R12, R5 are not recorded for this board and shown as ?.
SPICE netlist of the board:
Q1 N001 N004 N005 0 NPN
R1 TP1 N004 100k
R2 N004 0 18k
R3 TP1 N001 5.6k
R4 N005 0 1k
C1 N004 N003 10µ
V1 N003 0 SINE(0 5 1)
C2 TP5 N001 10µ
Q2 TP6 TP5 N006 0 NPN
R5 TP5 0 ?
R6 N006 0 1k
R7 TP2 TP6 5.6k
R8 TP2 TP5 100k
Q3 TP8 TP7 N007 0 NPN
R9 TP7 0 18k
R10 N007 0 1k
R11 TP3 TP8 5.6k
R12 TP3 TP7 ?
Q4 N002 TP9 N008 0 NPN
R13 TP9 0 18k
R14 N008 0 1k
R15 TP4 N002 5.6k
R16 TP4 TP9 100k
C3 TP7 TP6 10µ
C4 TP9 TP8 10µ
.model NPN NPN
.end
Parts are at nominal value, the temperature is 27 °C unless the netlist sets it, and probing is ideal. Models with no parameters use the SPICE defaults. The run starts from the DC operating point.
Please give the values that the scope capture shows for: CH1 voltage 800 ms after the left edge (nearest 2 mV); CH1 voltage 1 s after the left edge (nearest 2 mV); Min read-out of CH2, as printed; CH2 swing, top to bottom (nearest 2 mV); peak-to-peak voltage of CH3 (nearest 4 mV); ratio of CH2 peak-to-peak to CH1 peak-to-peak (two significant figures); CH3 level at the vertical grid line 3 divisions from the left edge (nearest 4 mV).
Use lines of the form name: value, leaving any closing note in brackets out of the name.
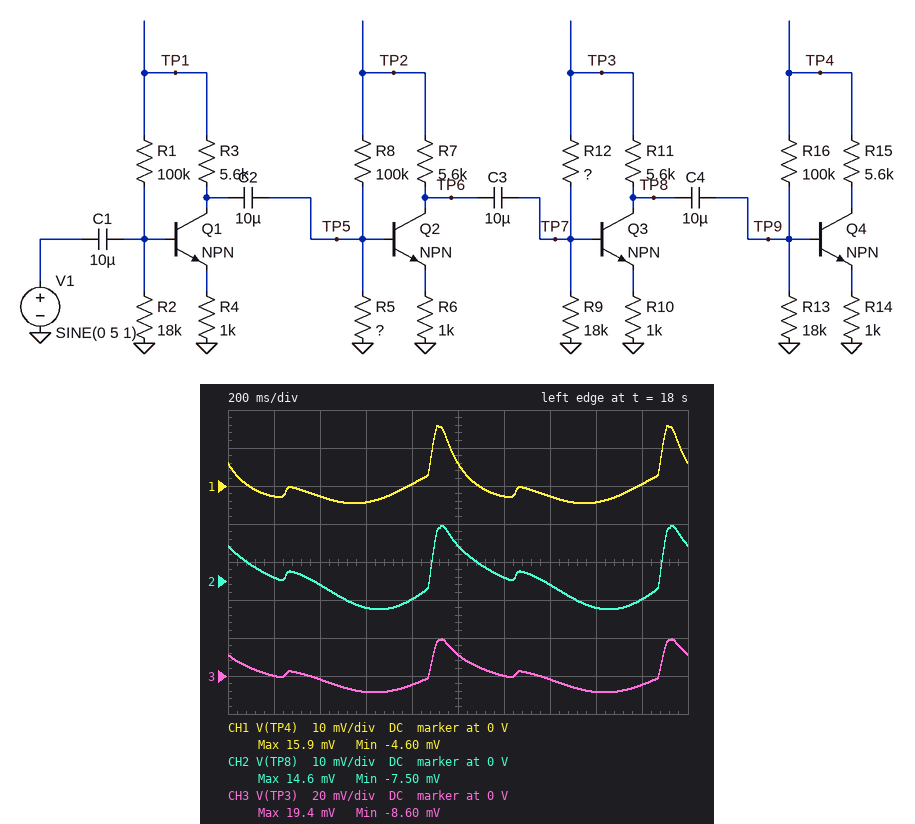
CH1 voltage 800 ms after the left edge: 0 V
CH1 voltage 1 s after the left edge: 6 mV
Min read-out of CH2, as printed: -7.50 mV
CH2 swing, top to bottom: 22 mV
peak-to-peak voltage of CH3: 28 mV
ratio of CH2 peak-to-peak to CH1 peak-to-peak: 1.1
CH3 level at the vertical grid line 3 divisions from the left edge: -8 mV
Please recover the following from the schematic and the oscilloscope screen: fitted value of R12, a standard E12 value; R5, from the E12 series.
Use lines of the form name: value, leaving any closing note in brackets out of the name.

fitted value of R12, a standard E12 value: 56 kΩ
R5, from the E12 series: 6.8 kΩ
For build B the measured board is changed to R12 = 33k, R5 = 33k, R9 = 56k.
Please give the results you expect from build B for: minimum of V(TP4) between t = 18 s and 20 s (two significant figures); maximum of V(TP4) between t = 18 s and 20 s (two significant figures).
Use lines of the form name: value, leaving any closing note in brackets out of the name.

minimum of V(TP4) between t = 18 s and 20 s: -38 mV
maximum of V(TP4) between t = 18 s and 20 s: 62 mV
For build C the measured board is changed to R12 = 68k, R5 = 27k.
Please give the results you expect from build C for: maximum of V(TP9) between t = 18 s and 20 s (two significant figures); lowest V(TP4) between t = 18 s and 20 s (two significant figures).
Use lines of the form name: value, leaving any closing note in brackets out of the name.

maximum of V(TP9) between t = 18 s and 20 s: 28 mV
lowest V(TP4) between t = 18 s and 20 s: -12 mV
